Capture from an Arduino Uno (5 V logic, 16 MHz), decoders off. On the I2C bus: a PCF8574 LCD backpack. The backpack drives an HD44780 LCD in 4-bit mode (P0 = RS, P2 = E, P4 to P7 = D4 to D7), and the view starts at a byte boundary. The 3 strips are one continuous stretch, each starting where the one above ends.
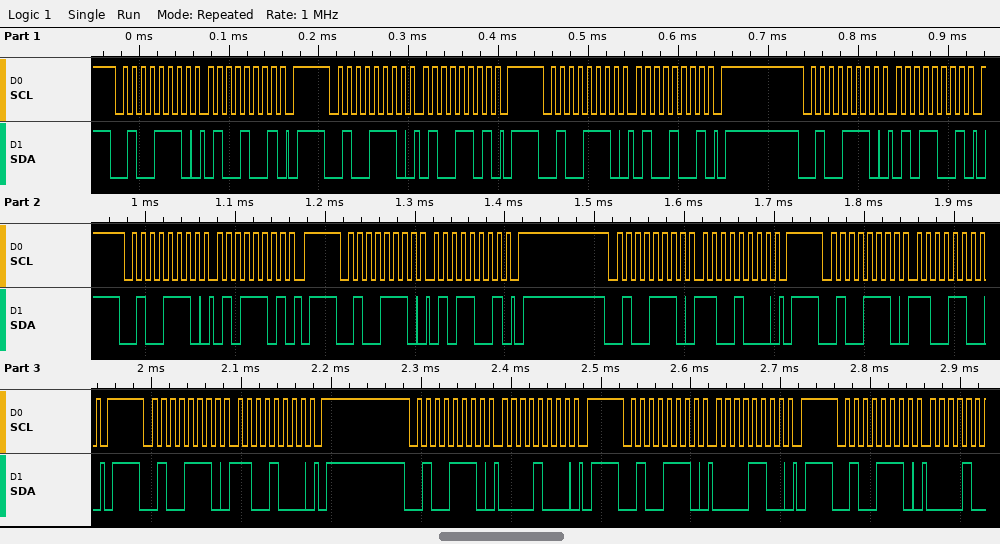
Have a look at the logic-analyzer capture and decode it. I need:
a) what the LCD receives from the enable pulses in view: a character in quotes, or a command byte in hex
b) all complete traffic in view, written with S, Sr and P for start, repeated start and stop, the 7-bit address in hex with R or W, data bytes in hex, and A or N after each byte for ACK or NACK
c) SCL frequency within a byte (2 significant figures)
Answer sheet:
'E'
S 27W A 49 A P S 27W A 4D A P S 27W A 49 A P S 27W A 59 A P S 27W A 5D A P S 27W A 59 A P S 27W A C8 A P S 27W A CC A P S 27W A C8 A P S 27W A 08 A P S 27W A 0C A P S 27W A
100 kHz
